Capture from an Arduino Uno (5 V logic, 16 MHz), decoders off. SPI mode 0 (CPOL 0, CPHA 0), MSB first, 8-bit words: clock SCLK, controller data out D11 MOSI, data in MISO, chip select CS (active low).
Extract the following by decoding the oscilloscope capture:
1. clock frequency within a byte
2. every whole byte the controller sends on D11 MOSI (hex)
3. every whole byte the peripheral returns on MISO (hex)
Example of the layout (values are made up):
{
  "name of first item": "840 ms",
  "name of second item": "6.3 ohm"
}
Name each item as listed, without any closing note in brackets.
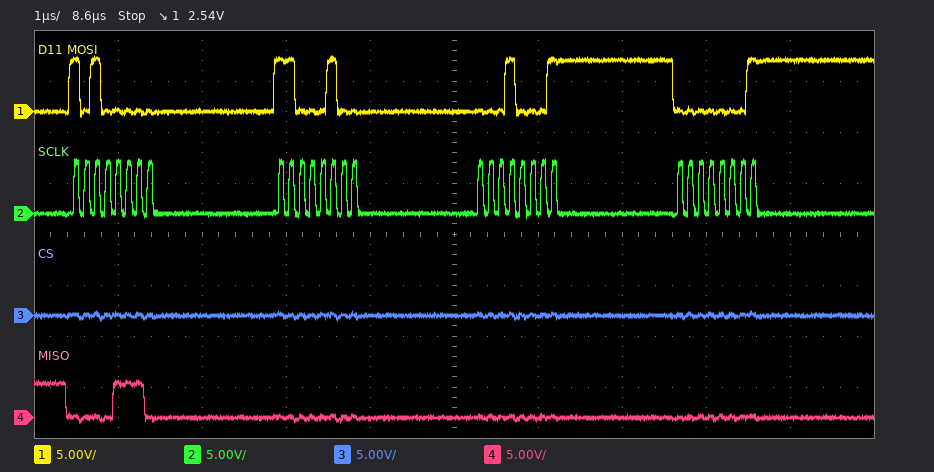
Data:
{
  "clock frequency within a byte": "8 MHz",
  "every whole byte the controller sends on D11 MOSI": "A0 C4 11 01",
  "every whole byte the peripheral returns on MISO": "0E 00 00 00"
}
